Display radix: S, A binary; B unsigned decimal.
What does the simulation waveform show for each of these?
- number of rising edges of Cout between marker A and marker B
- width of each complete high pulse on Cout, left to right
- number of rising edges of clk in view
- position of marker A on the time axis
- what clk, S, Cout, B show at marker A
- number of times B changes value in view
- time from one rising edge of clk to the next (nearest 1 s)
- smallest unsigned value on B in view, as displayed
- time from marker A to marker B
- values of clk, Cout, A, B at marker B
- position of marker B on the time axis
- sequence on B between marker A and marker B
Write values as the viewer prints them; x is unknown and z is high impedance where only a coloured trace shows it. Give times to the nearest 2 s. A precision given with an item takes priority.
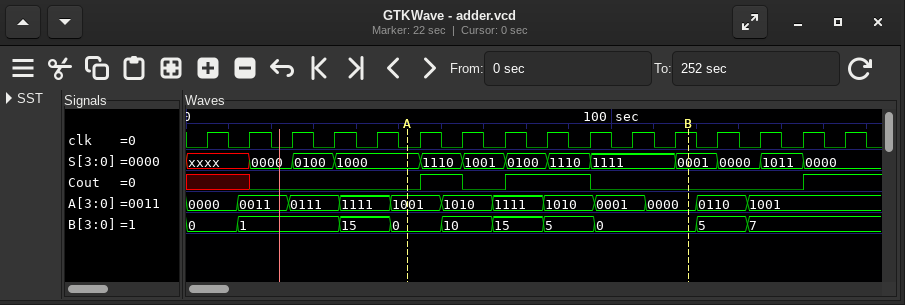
2
10 s, 20 s
16
52 s
clk=0, S=1000, Cout=0, B=0
9
10 s
0
66 s
clk=1, Cout=0, A=0000, B=0
118 s
0, 10, 15, 5, 0
